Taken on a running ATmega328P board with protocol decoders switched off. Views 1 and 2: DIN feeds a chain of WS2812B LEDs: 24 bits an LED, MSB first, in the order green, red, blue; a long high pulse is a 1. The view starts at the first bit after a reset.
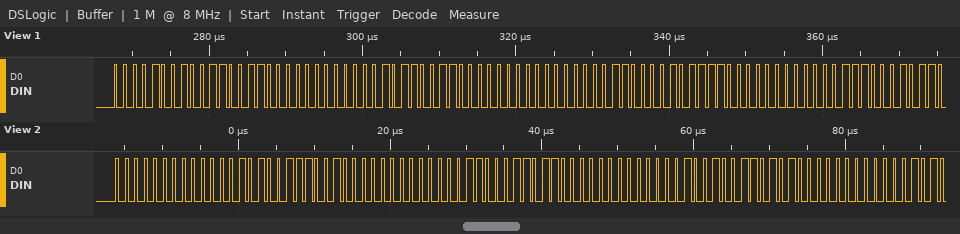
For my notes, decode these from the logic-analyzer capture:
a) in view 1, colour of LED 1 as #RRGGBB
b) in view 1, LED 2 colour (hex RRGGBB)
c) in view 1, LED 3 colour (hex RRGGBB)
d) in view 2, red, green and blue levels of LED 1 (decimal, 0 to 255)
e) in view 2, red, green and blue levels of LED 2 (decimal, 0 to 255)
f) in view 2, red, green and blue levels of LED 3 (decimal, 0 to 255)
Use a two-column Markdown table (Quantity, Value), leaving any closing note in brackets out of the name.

| Quantity | Value |
|---|---|
| in view 1, colour of LED 1 as #RRGGBB | #330900 |
| in view 1, LED 2 colour | #300B00 |
| in view 1, LED 3 colour | #2F0C00 |
| in view 2, red, green and blue levels of LED 1 | 5, 0, 57 |
| in view 2, red, green and blue levels of LED 2 | 6, 0, 54 |
| in view 2, red, green and blue levels of LED 3 | 9, 0, 53 |
